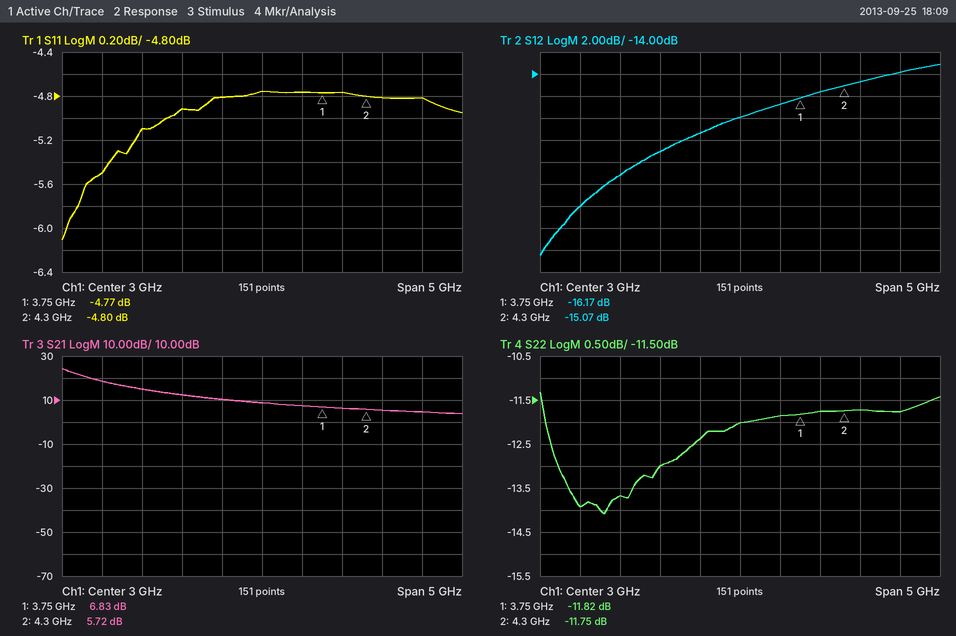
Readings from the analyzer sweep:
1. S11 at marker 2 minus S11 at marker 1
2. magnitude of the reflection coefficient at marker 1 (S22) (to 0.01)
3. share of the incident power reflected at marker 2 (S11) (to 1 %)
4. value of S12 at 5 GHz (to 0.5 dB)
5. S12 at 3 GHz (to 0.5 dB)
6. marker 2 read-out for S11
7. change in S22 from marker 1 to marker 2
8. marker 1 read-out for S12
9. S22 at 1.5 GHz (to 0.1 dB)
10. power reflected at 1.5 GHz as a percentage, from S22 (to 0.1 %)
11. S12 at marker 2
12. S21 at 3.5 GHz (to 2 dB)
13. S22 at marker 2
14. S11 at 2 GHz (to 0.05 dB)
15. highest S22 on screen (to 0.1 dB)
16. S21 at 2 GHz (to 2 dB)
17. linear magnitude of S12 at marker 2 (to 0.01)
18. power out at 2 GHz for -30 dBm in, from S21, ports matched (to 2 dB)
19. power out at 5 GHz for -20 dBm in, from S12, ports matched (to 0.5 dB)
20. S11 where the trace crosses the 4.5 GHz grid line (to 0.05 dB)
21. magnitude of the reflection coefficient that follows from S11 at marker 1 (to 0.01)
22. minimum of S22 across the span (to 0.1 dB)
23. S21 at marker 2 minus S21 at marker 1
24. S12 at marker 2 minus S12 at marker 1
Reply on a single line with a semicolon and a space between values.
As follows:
-0.03 dB; 0.26; 33 %; -14.0 dB; -18.0 dB; -4.80 dB; 0.07 dB; -16.17 dB; -13.7 dB; 4.3 %; -15.07 dB; 8 dB; -11.75 dB; -4.90 dB; -11.3 dB; 12 dB; 0.18; -18 dBm; -34.0 dBm; -4.80 dB; 0.58; -14.1 dB; -1.11 dB; 1.10 dB
